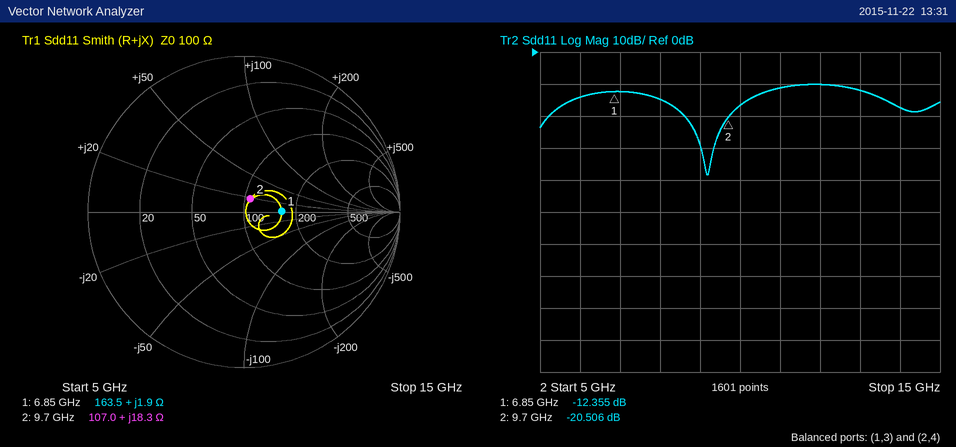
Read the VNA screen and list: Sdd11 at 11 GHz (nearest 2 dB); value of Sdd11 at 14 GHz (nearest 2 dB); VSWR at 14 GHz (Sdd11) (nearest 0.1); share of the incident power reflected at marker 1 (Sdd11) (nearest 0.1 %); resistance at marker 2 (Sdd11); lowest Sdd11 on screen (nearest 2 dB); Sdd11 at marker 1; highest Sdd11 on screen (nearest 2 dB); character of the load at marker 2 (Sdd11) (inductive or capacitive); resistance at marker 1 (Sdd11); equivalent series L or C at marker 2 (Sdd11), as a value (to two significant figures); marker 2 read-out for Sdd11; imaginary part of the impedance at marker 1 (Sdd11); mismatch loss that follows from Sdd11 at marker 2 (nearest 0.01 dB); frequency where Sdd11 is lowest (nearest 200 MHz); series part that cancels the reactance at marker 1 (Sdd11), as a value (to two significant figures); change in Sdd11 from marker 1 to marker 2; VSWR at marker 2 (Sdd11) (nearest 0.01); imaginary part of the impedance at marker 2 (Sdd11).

-12 dB
-18 dB
1.3
5.8 %
107.0 Ω
-38 dB
-12.355 dB
-10 dB
inductive
163.5 Ω
300 pH
-20.506 dB
+1.9 Ω
0.04 dB
9.2 GHz
12 pF
-8.151 dB
1.21
+18.3 Ω
